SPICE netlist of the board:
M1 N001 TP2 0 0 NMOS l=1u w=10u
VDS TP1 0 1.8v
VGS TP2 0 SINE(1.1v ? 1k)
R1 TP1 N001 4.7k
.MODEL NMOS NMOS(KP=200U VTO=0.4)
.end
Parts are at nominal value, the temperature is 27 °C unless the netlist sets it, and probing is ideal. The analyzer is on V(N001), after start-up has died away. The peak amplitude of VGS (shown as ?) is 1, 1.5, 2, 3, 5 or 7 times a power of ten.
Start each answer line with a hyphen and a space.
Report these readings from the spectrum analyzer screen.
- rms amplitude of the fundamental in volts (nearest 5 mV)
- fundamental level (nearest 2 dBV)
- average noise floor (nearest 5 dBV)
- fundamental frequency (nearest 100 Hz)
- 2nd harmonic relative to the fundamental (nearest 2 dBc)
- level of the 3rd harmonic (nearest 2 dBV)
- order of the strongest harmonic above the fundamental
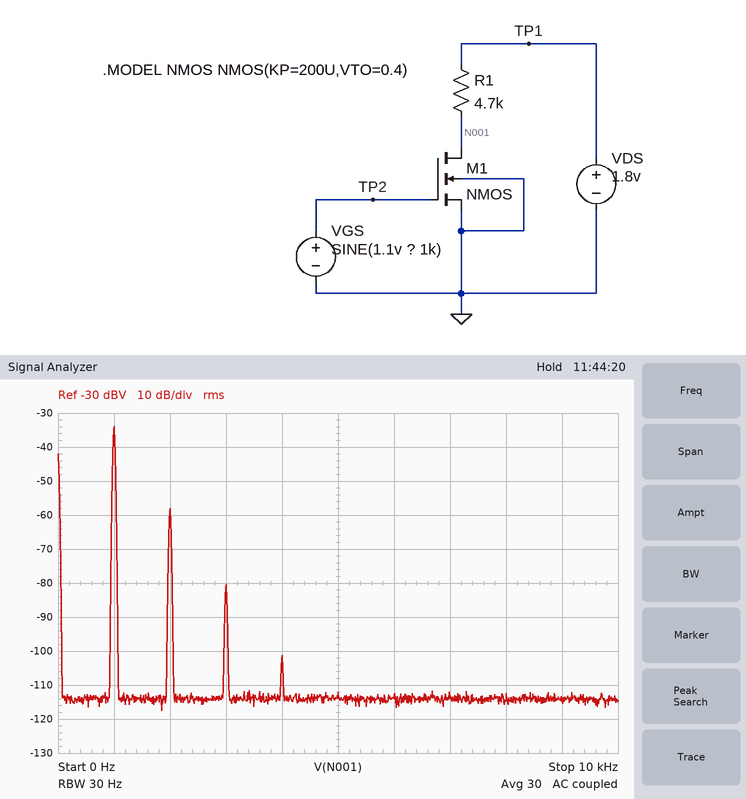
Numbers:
- 20 mV
- -34 dBV
- -115 dBV
- 1.0 kHz
- -24 dBc
- -80 dBV
- 2
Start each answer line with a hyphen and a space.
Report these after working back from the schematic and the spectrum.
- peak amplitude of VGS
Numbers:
- 50 mV
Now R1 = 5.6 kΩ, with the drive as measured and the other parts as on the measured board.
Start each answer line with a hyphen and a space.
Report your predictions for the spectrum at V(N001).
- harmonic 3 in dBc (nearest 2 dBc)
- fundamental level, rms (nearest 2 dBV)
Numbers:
- -48 dBc
- -36 dBV
